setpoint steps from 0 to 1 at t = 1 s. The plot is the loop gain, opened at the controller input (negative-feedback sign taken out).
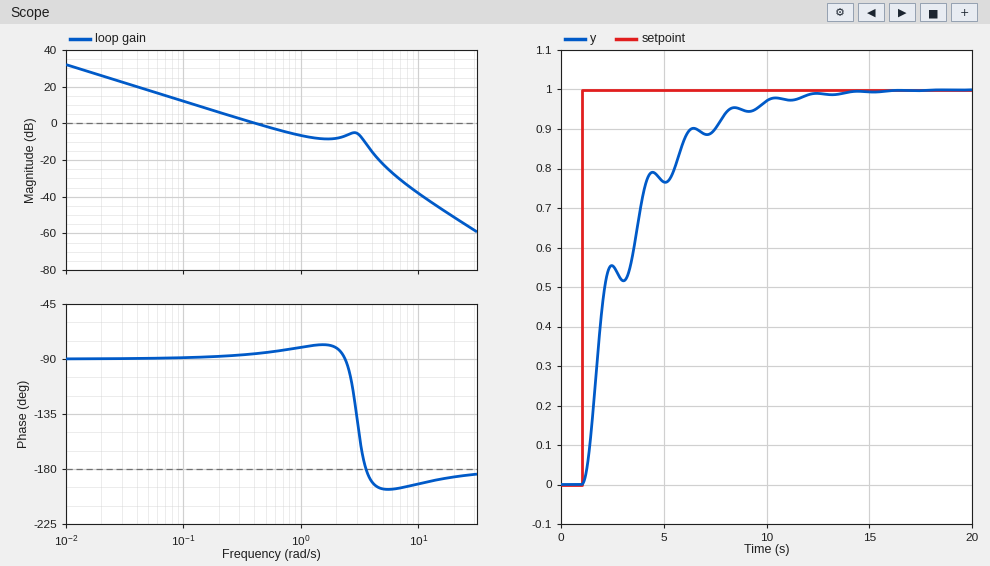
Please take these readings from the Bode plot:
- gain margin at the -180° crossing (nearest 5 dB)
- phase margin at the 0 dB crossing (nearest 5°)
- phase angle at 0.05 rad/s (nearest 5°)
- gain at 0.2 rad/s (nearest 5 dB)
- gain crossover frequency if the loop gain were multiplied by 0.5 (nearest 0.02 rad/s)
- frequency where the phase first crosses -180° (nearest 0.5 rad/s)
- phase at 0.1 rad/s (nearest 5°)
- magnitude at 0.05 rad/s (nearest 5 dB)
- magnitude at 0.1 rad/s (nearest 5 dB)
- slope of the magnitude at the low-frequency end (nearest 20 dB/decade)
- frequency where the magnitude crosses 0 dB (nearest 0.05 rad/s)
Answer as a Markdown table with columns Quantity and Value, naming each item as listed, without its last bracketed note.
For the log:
| Quantity | Value |
|---|---|
| gain margin at the -180° crossing | 10 dB |
| phase margin at the 0 dB crossing | 95° |
| phase angle at 0.05 rad/s | -90° |
| gain at 0.2 rad/s | 5 dB |
| gain crossover frequency if the loop gain were multiplied by 0.5 | 0.20 rad/s |
| frequency where the phase first crosses -180° | 3.5 rad/s |
| phase at 0.1 rad/s | -90° |
| magnitude at 0.05 rad/s | 20 dB |
| magnitude at 0.1 rad/s | 10 dB |
| slope of the magnitude at the low-frequency end | -20 dB/decade |
| frequency where the magnitude crosses 0 dB | 0.40 rad/s |
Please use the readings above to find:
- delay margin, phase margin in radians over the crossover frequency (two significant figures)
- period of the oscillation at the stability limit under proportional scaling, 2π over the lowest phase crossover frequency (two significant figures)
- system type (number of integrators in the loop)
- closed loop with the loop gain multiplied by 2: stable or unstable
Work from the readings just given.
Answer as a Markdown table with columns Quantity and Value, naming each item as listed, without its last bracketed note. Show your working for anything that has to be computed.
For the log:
| Quantity | Value |
|---|---|
| delay margin, phase margin in radians over the crossover frequency | 95 × π / 180 / 0.4 = 4.1 s |
| period of the oscillation at the stability limit under proportional scaling, 2π over the lowest phase crossover frequency | 2π / 3.5 = 1.8 s |
| system type | 1 |
| closed loop with the loop gain multiplied by 2: stable or unstable | stable |
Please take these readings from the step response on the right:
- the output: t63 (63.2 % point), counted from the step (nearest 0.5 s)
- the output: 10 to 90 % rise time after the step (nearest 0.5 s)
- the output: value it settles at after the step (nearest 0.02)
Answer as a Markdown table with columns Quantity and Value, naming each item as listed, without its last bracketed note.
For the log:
| Quantity | Value |
|---|---|
| the output: t63 (63.2 % point), counted from the step | 2.5 s |
| the output: 10 to 90 % rise time after the step | 5.0 s |
| the output: value it settles at after the step | 1.00 |
